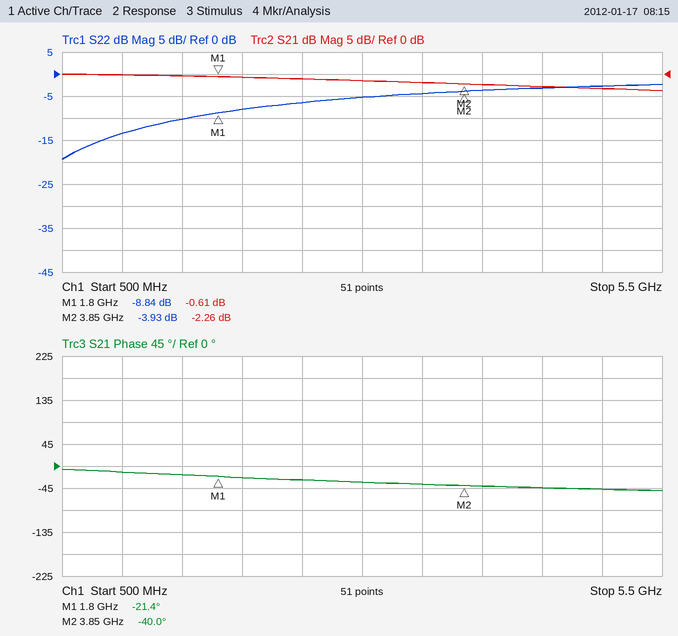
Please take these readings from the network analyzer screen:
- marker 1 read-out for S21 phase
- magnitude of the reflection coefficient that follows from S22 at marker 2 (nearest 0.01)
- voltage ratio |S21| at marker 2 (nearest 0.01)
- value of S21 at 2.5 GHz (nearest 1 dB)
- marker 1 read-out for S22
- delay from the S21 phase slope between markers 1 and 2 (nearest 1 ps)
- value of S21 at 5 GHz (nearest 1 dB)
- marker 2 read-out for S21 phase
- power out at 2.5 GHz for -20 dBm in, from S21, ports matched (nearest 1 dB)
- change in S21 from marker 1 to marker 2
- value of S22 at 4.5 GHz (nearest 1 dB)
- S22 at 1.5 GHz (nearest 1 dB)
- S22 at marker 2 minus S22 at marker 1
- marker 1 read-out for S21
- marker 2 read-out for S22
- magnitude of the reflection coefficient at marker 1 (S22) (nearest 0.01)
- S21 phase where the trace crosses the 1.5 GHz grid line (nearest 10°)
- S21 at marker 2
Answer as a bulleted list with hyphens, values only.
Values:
- -21.4°
- 0.64
- 0.77
- -1 dB
- -8.84 dB
- 25 ps
- -3 dB
- -40.0°
- -21 dBm
- -1.65 dB
- -3 dB
- -10 dB
- 4.91 dB
- -0.61 dB
- -3.93 dB
- 0.36
- -20°
- -2.26 dB
